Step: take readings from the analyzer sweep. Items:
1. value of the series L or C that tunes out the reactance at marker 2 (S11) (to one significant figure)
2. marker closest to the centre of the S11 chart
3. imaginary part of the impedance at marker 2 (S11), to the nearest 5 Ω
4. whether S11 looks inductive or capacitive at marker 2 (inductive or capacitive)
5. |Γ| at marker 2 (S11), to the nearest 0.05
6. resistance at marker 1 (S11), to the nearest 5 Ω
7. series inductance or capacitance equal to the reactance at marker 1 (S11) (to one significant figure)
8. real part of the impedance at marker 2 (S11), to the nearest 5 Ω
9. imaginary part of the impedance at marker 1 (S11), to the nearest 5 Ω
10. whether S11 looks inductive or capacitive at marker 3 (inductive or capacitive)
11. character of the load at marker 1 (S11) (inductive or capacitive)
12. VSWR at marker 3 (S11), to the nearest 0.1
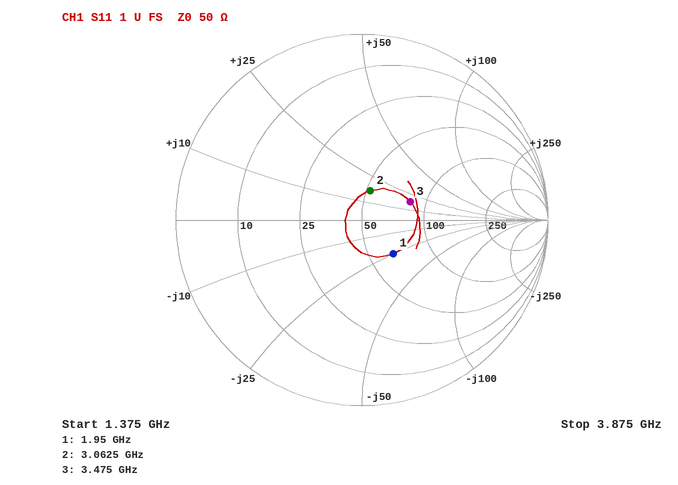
3 pF
marker 2
+15 Ω
inductive
0.15
65 Ω
3 pF
50 Ω
-25 Ω
inductive
capacitive
1.8
